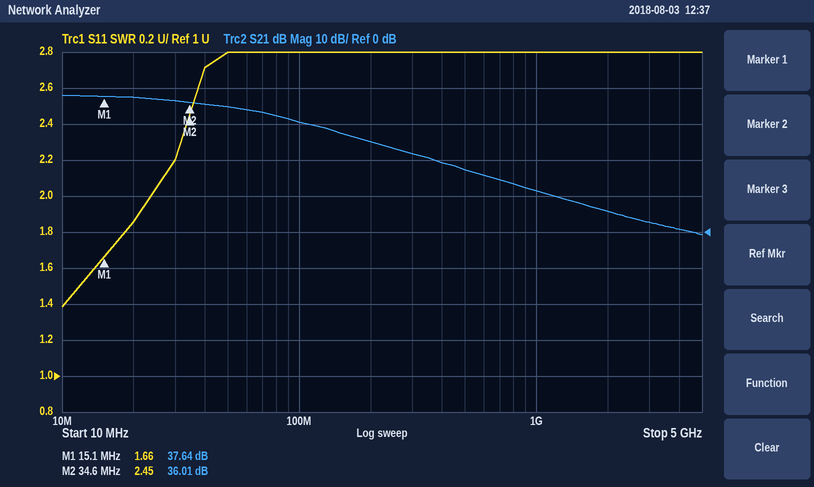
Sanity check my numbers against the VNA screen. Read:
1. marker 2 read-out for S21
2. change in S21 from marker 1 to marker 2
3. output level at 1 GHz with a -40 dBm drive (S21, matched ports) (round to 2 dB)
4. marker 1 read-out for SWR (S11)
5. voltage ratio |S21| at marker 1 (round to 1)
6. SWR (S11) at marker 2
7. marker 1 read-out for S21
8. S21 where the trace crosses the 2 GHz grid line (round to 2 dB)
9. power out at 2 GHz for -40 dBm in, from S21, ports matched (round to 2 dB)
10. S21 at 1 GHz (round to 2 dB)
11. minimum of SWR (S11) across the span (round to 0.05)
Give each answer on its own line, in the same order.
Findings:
36.01 dB
-1.63 dB
-28 dBm
1.66
76
2.45
37.64 dB
6 dB
-34 dBm
12 dB
1.40
